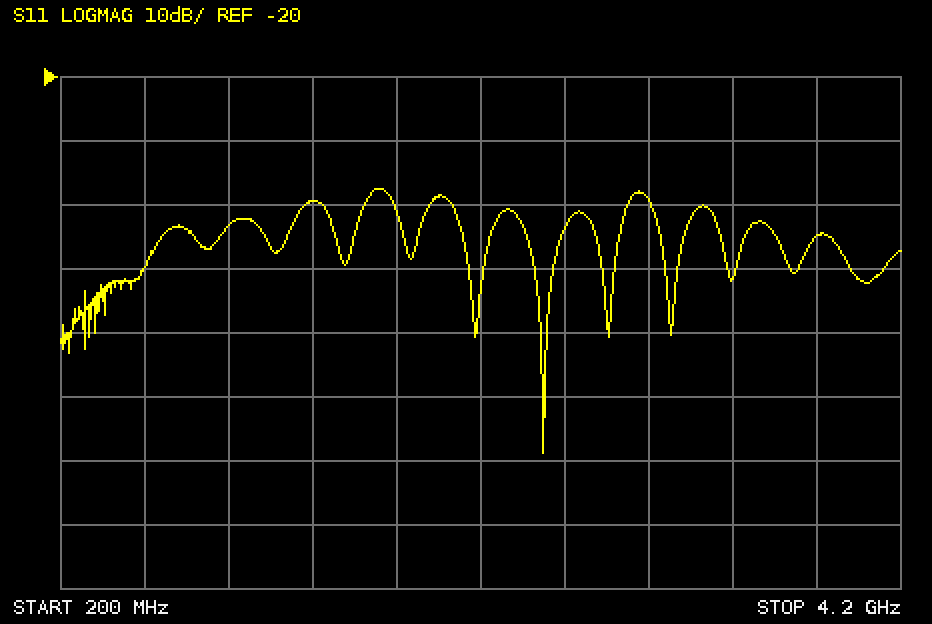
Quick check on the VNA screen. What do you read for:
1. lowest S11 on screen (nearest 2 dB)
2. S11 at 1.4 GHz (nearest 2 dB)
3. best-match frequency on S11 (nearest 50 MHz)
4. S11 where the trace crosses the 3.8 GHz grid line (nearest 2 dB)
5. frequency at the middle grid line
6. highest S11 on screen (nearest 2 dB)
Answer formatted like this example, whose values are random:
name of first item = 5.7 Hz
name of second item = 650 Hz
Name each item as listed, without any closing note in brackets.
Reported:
lowest S11 on screen = -78 dB
S11 at 1.4 GHz = -40 dB
best-match frequency on S11 = 2.50 GHz
S11 where the trace crosses the 3.8 GHz grid line = -44 dB
frequency at the middle grid line = 2.2 GHz
highest S11 on screen = -38 dB
